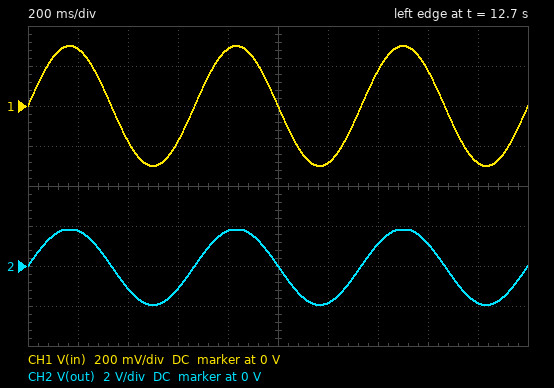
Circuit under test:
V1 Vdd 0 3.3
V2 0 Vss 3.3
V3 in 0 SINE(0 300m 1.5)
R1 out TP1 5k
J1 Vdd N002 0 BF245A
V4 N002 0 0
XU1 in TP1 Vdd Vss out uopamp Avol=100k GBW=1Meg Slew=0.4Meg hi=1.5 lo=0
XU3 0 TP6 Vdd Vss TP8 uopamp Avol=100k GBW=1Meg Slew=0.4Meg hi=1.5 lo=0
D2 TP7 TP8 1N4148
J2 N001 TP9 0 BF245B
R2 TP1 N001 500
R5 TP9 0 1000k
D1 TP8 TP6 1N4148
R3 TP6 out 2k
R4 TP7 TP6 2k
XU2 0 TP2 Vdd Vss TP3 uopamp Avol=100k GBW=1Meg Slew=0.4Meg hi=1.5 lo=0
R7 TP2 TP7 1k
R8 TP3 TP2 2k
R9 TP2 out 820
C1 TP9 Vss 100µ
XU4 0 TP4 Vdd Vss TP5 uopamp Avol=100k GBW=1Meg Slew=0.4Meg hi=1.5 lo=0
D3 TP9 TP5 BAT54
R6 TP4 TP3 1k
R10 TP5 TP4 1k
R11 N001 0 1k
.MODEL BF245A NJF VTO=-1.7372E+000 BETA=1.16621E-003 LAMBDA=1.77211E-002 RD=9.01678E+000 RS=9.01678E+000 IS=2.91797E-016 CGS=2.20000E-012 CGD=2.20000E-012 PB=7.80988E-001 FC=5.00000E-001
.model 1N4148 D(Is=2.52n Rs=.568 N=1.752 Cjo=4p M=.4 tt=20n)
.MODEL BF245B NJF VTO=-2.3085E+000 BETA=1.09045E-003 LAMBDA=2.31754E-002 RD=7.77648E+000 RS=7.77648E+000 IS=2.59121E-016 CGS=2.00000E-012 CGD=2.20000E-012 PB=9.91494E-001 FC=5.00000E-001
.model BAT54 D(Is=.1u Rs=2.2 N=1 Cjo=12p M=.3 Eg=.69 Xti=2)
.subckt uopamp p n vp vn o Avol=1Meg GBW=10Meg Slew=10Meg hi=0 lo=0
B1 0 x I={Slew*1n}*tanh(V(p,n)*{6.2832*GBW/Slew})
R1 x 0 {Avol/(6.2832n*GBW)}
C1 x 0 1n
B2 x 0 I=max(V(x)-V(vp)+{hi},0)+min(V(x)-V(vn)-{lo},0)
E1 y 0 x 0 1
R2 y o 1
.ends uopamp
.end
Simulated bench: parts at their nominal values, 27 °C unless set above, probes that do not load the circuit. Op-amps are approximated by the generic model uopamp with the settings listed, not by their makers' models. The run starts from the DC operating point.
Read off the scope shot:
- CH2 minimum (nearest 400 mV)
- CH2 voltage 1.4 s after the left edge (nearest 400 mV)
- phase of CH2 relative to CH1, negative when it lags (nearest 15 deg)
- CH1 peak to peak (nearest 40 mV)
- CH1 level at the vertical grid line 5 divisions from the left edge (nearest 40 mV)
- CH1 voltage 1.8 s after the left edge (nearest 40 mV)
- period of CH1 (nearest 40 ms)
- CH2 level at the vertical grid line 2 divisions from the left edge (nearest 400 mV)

-2.0 V
1.2 V
0 deg
600 mV
0 V
-280 mV
680 ms
-1.2 V
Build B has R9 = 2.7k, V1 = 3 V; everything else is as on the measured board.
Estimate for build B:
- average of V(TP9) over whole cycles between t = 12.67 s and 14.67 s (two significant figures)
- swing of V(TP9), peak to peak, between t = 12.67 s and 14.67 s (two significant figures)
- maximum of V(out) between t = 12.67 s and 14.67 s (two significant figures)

-1.4 V
4.3 mV
1.5 V
